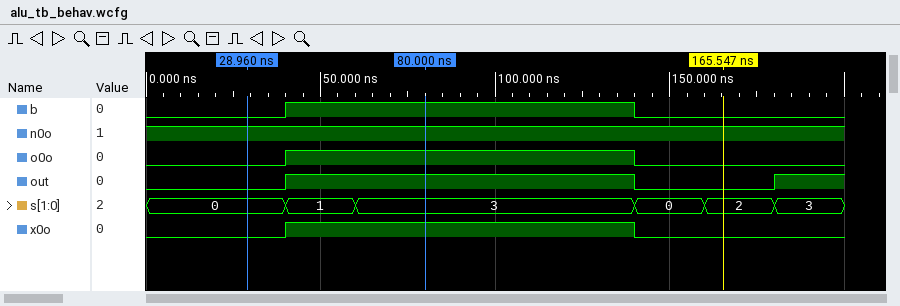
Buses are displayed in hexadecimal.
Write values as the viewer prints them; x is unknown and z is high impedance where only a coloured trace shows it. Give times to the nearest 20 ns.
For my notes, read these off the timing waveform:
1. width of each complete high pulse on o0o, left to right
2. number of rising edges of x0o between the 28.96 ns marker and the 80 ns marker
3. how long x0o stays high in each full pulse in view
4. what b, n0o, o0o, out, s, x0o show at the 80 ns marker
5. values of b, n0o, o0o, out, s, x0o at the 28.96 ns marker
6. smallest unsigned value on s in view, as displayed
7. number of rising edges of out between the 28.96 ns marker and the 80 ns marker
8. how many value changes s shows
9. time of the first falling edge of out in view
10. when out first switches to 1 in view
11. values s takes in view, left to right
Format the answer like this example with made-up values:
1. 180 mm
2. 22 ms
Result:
1. 100 ns
2. 1
3. 100 ns
4. b=1, n0o=1, o0o=1, out=1, s=3, x0o=1
5. b=0, n0o=1, o0o=0, out=0, s=0, x0o=0
6. 0
7. 1
8. 5
9. 140 ns
10. 40 ns
11. 0, 1, 3, 0, 2, 3
